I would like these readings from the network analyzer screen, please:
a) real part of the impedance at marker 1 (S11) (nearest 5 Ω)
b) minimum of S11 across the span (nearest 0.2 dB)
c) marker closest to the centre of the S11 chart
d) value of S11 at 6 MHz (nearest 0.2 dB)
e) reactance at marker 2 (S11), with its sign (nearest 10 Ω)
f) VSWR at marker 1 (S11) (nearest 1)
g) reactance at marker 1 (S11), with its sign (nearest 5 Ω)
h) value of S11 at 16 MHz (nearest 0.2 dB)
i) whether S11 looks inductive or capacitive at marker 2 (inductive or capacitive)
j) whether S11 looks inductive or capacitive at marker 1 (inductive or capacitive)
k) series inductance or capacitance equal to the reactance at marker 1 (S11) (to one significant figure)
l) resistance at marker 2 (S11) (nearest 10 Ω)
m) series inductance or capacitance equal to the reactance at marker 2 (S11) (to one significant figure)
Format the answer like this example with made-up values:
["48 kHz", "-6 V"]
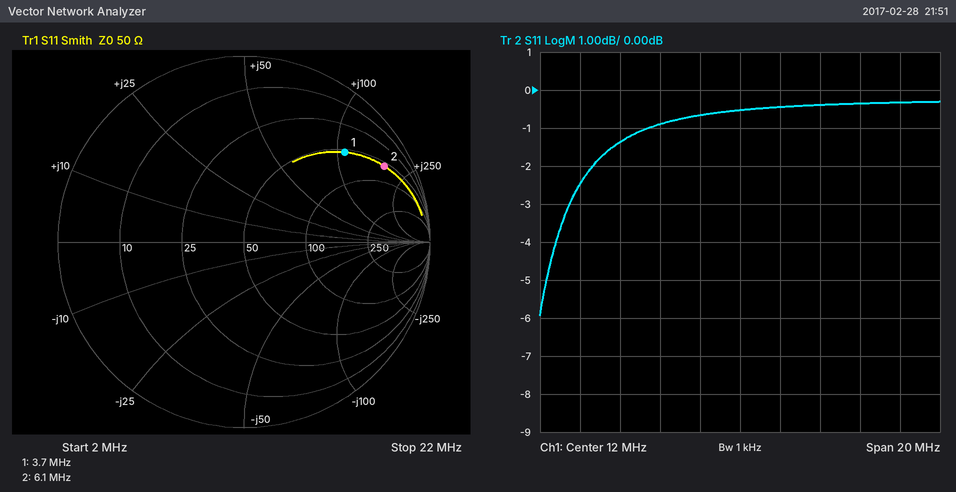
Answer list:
["55 Ω", "-6.0 dB", "marker 1", "-1.4 dB", "+180 Ω", "6", "+110 Ω", "-0.4 dB", "inductive", "inductive", "5 µH", "60 Ω", "5 µH"]
